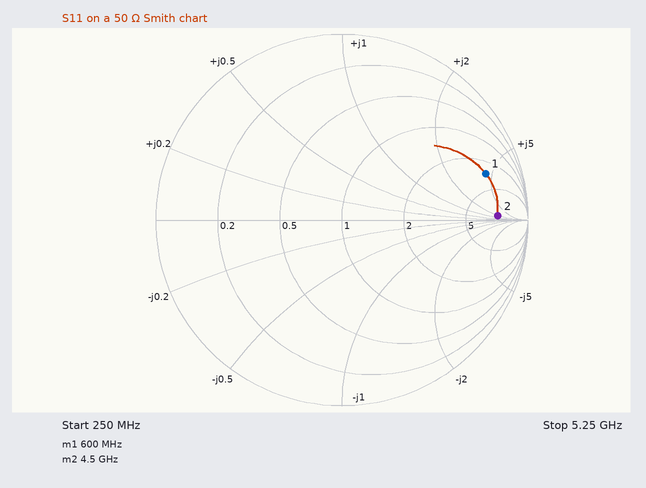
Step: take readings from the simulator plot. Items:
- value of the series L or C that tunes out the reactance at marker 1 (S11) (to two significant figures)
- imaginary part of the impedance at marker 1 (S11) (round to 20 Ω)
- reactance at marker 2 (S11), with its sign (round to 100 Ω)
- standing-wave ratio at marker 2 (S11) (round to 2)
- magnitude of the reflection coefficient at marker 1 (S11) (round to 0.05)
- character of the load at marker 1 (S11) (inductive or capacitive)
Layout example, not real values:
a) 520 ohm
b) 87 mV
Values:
a) 1.2 pF
b) +220 Ω
c) +100 Ω
d) 12
e) 0.80
f) inductive
